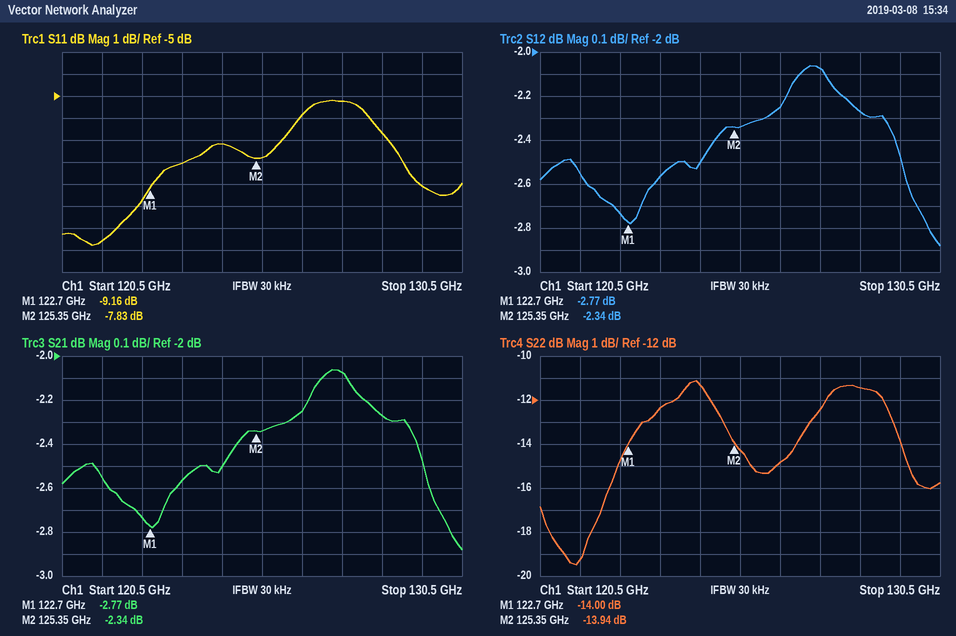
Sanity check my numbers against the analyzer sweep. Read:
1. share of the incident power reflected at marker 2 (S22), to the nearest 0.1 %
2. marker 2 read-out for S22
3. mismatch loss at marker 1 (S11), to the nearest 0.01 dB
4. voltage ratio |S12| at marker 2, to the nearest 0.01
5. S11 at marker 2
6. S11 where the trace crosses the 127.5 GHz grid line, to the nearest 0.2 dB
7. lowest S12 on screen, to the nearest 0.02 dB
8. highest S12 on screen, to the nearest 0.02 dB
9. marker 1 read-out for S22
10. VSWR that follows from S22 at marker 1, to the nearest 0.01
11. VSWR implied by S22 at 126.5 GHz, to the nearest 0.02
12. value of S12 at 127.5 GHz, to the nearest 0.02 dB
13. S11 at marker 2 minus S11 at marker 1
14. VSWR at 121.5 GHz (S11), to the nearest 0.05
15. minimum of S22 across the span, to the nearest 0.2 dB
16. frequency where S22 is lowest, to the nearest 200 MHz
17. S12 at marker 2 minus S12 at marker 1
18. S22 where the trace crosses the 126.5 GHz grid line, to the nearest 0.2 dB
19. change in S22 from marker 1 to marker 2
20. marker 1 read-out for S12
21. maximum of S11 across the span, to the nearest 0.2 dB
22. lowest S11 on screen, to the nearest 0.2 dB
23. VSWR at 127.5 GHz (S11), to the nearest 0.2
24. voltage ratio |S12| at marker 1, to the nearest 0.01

4.0 %
-13.94 dB
0.56 dB
0.76
-7.83 dB
-5.2 dB
-2.88 dB
-2.06 dB
-14.00 dB
1.50
1.44
-2.08 dB
1.33 dB
1.70
-19.4 dB
121.4 GHz
0.43 dB
-14.8 dB
0.06 dB
-2.77 dB
-5.2 dB
-11.8 dB
3.4
0.73
